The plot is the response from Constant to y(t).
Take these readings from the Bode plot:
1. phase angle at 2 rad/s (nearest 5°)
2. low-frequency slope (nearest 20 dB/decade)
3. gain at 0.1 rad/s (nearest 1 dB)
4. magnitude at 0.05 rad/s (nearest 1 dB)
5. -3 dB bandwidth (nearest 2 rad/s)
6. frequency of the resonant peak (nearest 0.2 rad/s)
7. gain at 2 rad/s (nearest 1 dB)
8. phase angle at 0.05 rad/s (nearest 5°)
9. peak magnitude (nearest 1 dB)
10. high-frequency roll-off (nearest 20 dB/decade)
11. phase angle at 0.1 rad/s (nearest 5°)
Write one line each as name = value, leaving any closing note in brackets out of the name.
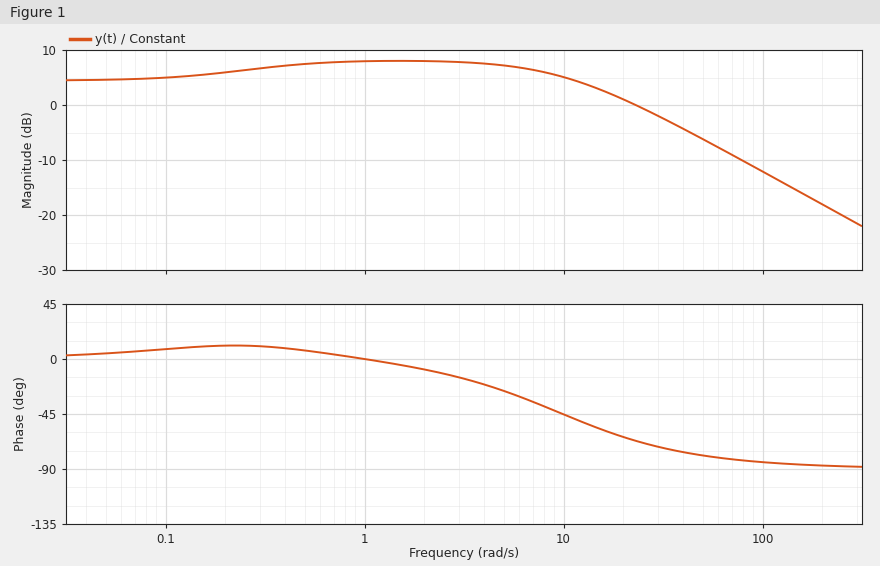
phase angle at 2 rad/s = -10°
low-frequency slope = 0 dB/decade
gain at 0.1 rad/s = 5 dB
magnitude at 0.05 rad/s = 5 dB
-3 dB bandwidth = 18 rad/s
frequency of the resonant peak = 1.4 rad/s
gain at 2 rad/s = 8 dB
phase angle at 0.05 rad/s = 5°
peak magnitude = 8 dB
high-frequency roll-off = -20 dB/decade
phase angle at 0.1 rad/s = 10°
